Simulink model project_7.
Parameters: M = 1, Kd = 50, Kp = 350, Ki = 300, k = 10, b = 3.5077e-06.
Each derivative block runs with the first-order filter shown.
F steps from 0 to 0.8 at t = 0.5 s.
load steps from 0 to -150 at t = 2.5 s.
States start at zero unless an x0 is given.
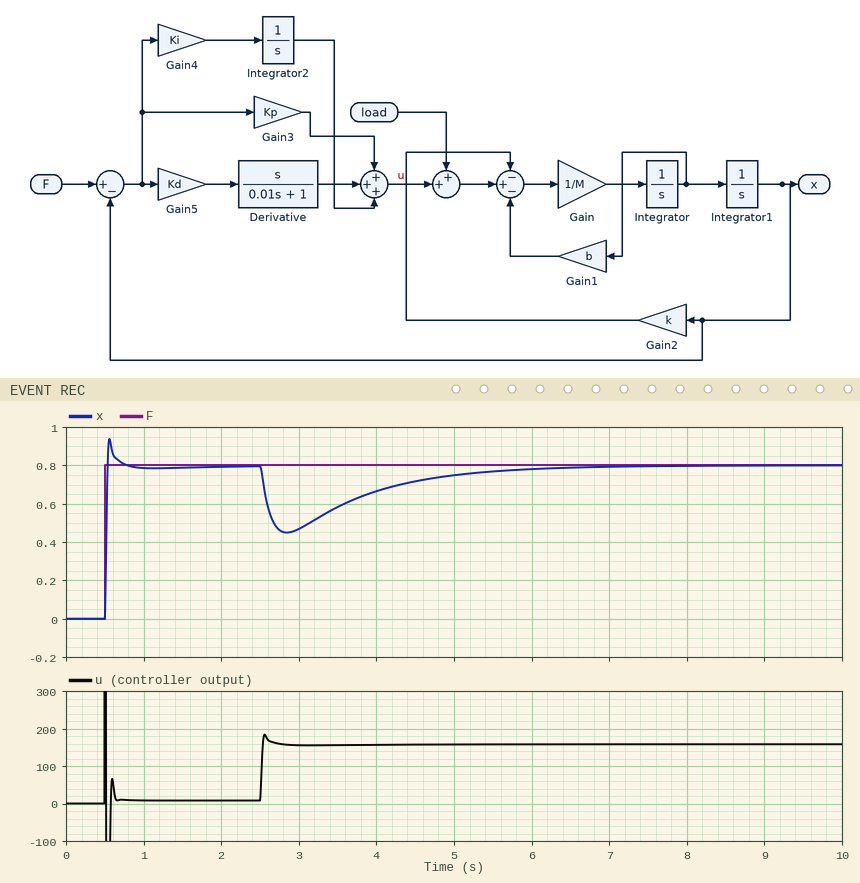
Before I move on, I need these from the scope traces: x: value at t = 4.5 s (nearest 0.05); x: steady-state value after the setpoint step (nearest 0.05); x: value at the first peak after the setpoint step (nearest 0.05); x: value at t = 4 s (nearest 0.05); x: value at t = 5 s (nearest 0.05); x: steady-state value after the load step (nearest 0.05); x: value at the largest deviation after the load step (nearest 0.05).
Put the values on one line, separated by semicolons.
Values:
0.70; 0.80; 0.95; 0.65; 0.75; 0.80; 0.45
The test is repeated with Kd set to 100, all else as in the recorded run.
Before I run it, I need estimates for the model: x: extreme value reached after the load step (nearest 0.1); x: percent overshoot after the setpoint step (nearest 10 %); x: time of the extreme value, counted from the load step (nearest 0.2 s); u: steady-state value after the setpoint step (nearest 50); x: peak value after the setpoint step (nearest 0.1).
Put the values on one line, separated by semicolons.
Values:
0.5; 20 %; 0.6 s; 0; 1.0
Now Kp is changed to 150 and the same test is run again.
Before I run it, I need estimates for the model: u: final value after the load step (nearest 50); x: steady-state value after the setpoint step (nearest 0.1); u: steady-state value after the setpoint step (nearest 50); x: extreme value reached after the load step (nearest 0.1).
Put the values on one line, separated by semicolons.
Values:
150; 0.8; 0; 0.2
